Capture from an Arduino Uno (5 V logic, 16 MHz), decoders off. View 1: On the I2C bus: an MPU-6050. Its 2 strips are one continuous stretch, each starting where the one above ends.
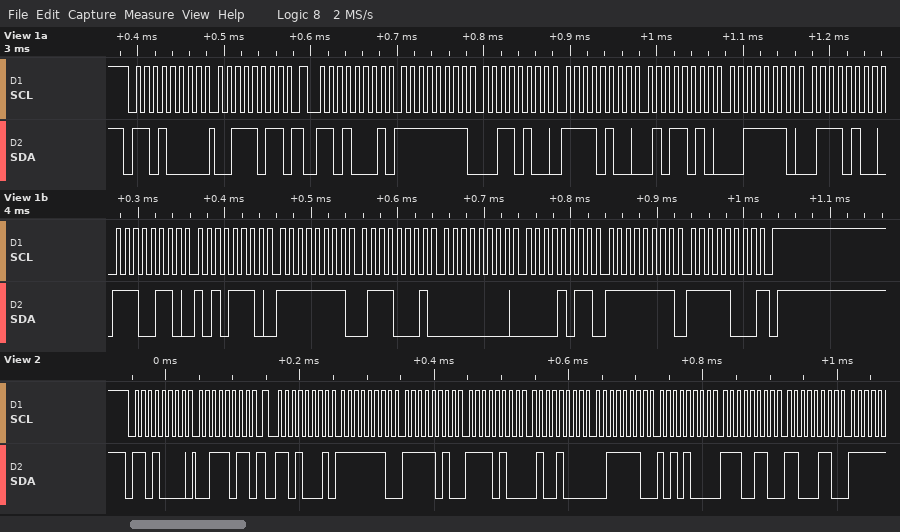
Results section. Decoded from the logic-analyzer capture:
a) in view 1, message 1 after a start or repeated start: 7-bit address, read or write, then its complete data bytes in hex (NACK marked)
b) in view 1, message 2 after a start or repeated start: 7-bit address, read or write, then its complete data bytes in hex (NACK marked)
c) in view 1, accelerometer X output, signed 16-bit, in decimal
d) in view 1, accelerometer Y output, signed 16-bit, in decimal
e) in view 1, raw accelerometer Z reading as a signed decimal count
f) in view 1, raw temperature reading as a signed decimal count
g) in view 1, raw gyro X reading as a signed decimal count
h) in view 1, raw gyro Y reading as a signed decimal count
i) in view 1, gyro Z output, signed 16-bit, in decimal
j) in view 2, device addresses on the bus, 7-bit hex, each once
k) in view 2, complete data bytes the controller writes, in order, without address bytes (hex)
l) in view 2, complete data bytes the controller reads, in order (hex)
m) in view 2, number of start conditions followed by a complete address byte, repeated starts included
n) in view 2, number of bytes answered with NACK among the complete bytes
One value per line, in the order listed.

0x68 write: 3B
0x68 read: FF 34 F4 5A 3E 74 E6 AE FF 71 00 0B FF F8 NACK
-204
-2982
15988
-6482
-143
11
-8
0x68
3B
FE FA F4 48 3E A8 E6 C6
2
0
